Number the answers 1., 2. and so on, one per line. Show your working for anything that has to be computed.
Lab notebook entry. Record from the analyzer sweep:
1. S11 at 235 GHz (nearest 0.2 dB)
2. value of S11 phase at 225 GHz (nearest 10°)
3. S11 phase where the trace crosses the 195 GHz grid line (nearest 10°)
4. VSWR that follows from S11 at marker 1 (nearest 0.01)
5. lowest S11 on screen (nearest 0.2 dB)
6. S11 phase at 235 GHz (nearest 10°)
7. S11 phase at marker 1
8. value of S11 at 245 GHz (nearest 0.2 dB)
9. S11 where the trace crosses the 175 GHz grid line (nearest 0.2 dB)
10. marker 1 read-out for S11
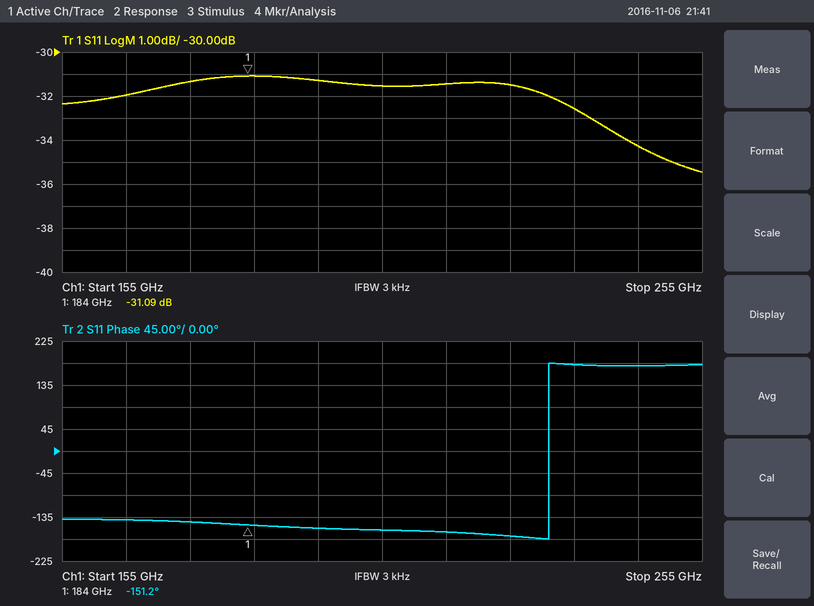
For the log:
1. -32.6 dB
2. -170°
3. -160°
4. (1 + 0.0279)/(1 − 0.0279) ≈ 1.06
5. -35.4 dB
6. 180°
7. -151.2°
8. -34.2 dB
9. -31.4 dB
10. -31.09 dB
